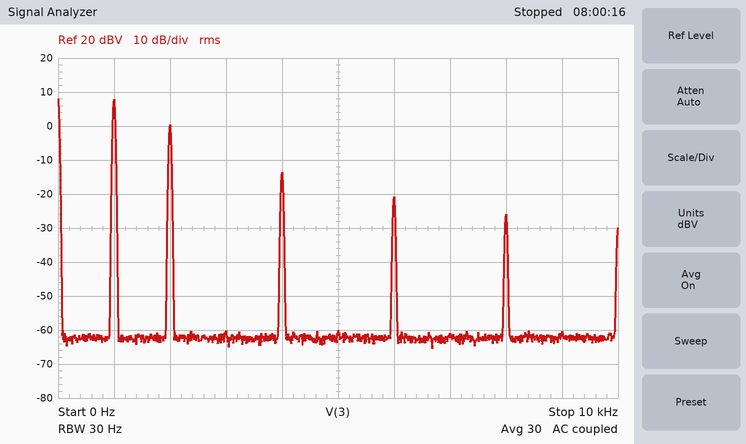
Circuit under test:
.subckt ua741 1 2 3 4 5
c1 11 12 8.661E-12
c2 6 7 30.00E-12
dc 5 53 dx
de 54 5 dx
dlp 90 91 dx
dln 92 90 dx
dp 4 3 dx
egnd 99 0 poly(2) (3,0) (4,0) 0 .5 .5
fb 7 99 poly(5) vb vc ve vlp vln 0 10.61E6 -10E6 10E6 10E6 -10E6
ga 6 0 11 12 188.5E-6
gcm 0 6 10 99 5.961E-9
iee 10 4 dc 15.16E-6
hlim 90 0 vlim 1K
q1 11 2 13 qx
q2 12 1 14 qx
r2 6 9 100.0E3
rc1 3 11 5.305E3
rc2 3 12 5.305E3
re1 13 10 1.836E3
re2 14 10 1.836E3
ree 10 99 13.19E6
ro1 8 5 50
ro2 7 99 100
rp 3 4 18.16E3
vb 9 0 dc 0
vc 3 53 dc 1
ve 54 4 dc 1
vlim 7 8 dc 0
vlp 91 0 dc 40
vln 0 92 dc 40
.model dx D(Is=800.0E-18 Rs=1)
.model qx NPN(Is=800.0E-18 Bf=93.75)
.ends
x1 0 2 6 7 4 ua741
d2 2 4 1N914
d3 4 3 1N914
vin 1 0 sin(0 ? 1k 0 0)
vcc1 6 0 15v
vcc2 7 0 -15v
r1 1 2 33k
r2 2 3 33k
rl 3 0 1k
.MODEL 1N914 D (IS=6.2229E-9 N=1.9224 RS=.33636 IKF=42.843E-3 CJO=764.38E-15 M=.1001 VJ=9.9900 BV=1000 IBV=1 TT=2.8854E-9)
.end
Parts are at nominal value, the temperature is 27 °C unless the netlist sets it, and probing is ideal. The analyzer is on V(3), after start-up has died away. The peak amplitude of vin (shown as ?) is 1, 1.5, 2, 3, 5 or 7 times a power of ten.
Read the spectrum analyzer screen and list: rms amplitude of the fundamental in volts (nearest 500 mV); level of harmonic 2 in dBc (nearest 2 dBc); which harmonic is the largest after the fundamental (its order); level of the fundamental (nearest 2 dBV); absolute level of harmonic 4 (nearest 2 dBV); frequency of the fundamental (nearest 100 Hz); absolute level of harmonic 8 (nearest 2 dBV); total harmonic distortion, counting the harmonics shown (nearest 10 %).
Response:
2.5 V
-8 dBc
2
8 dBV
-14 dBV
1.0 kHz
-26 dBV
40 %
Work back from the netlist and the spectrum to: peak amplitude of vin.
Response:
7 V
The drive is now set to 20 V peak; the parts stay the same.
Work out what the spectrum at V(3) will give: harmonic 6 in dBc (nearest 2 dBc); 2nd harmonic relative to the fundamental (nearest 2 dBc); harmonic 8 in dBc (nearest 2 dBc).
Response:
-26 dBc
-10 dBc
-42 dBc
